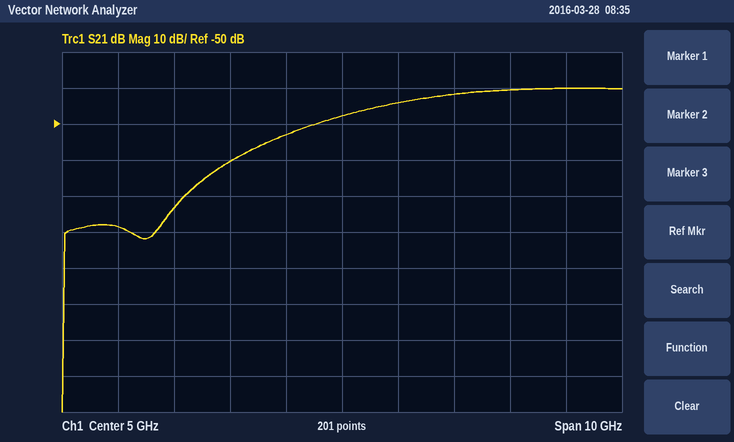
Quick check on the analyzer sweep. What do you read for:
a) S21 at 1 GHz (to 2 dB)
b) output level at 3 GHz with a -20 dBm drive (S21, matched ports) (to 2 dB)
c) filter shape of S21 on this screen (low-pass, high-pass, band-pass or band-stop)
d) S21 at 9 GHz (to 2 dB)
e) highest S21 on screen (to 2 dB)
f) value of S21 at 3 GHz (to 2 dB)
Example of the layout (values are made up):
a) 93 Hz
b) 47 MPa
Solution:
a) -78 dB
b) -80 dBm
c) high-pass
d) -40 dB
e) -40 dB
f) -60 dB
